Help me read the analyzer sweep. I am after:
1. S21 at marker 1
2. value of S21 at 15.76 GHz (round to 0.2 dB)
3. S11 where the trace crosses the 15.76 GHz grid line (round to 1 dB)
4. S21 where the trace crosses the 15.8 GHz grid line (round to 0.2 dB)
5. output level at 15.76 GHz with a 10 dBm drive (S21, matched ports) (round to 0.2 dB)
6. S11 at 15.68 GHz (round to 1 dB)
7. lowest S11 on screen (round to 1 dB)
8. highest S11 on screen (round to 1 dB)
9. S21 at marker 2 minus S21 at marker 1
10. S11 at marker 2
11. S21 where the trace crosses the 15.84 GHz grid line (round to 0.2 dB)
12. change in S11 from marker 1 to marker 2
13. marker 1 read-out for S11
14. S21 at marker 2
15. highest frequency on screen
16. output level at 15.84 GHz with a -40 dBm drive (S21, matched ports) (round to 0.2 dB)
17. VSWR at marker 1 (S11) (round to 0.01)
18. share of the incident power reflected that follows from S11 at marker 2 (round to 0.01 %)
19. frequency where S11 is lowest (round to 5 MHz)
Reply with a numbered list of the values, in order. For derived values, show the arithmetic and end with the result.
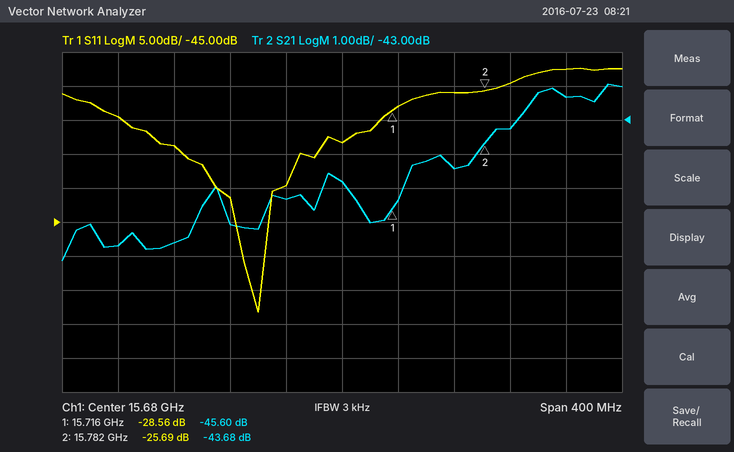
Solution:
1. -45.60 dB
2. -44.4 dB
3. -26 dB
4. -43.2 dB
5. 10 dBm + (-44.4 dB) = -34.4 dBm
6. -33 dB
7. -58 dB
8. -22 dB
9. -43.68 − (-45.6) = 1.92 dB
10. -25.69 dB
11. -42.4 dB
12. -25.69 − (-28.56) = 2.87 dB
13. -28.56 dB
14. -43.68 dB
15. 15.88 GHz
16. -40 dBm + (-42.4 dB) = -82.4 dBm
17. (1 + 0.0373)/(1 − 0.0373) ≈ 1.08
18. 10^(-25.69/10) ≈ 0.27 %
19. 15.620 GHz
